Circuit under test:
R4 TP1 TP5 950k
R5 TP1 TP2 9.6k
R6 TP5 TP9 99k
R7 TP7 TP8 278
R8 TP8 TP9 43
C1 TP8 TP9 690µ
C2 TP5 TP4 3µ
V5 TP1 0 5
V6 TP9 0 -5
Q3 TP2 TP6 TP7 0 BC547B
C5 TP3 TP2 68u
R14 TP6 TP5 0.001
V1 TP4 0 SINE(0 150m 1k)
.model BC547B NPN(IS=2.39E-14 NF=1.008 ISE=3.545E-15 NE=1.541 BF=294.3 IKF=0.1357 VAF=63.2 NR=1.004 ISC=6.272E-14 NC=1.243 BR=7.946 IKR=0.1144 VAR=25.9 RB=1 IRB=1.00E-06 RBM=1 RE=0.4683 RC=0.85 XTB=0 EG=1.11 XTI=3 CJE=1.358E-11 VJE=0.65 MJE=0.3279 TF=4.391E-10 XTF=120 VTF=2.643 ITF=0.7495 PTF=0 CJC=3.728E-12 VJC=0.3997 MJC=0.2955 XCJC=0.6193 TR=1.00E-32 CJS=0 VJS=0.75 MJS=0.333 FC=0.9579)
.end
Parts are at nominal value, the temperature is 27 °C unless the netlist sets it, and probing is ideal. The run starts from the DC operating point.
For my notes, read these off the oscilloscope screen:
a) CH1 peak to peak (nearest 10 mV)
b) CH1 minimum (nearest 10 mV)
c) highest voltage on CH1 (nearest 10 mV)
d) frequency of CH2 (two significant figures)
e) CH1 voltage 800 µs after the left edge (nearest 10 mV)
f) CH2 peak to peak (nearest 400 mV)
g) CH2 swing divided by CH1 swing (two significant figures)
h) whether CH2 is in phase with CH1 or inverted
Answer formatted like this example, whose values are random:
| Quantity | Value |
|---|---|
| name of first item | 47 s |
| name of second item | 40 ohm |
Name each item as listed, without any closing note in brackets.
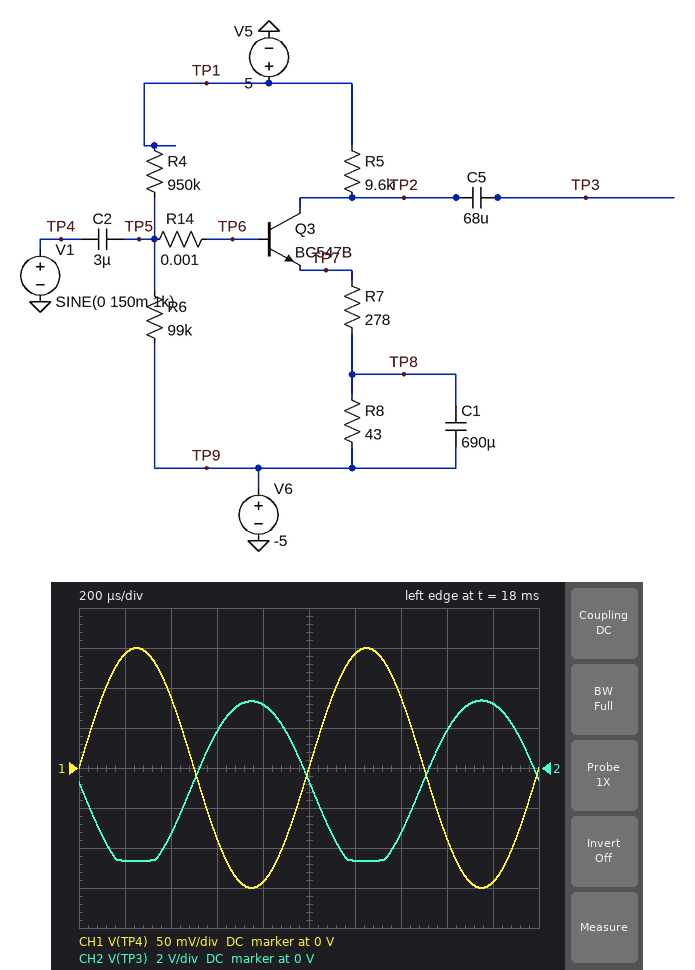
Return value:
| Quantity | Value |
|---|---|
| CH1 peak to peak | 300 mV |
| CH1 minimum | -150 mV |
| highest voltage on CH1 | 150 mV |
| frequency of CH2 | 1.0 kHz |
| CH1 voltage 800 µs after the left edge | -140 mV |
| CH2 peak to peak | 8.0 V |
| CH2 swing divided by CH1 swing | 27 |
| whether CH2 is in phase with CH1 or inverted | inverted |
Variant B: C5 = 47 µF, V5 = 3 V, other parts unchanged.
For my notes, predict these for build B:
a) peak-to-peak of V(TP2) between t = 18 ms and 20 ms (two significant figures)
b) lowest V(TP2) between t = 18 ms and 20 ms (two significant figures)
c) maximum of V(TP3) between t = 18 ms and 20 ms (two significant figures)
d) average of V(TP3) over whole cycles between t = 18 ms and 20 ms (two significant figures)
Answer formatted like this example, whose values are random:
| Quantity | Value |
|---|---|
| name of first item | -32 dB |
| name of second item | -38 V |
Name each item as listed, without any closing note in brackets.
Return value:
| Quantity | Value |
|---|---|
| peak-to-peak of V(TP2) between t = 18 ms and 20 ms | 7.2 V |
| lowest V(TP2) between t = 18 ms and 20 ms | -4.7 V |
| maximum of V(TP3) between t = 18 ms and 20 ms | 2.5 V |
| average of V(TP3) over whole cycles between t = 18 ms and 20 ms | -1.1 V |
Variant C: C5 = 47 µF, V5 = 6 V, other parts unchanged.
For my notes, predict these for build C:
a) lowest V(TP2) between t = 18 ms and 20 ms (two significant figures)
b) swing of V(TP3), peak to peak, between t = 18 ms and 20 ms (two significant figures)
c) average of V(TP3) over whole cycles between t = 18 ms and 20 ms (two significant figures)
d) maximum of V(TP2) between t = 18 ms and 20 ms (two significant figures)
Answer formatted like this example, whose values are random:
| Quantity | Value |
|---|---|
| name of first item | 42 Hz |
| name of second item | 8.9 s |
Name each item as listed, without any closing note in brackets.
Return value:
| Quantity | Value |
|---|---|
| lowest V(TP2) between t = 18 ms and 20 ms | -4.6 V |
| swing of V(TP3), peak to peak, between t = 18 ms and 20 ms | 8.3 V |
| average of V(TP3) over whole cycles between t = 18 ms and 20 ms | -590 mV |
| maximum of V(TP2) between t = 18 ms and 20 ms | 3.7 V |
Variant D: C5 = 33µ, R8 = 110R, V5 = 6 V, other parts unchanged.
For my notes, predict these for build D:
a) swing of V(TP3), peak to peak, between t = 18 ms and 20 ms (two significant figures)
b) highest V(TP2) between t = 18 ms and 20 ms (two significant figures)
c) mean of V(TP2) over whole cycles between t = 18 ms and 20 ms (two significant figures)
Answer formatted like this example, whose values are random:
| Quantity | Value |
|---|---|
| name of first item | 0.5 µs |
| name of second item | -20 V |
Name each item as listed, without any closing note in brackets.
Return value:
| Quantity | Value |
|---|---|
| swing of V(TP3), peak to peak, between t = 18 ms and 20 ms | 8.3 V |
| highest V(TP2) between t = 18 ms and 20 ms | 3.7 V |
| mean of V(TP2) over whole cycles between t = 18 ms and 20 ms | -530 mV |
